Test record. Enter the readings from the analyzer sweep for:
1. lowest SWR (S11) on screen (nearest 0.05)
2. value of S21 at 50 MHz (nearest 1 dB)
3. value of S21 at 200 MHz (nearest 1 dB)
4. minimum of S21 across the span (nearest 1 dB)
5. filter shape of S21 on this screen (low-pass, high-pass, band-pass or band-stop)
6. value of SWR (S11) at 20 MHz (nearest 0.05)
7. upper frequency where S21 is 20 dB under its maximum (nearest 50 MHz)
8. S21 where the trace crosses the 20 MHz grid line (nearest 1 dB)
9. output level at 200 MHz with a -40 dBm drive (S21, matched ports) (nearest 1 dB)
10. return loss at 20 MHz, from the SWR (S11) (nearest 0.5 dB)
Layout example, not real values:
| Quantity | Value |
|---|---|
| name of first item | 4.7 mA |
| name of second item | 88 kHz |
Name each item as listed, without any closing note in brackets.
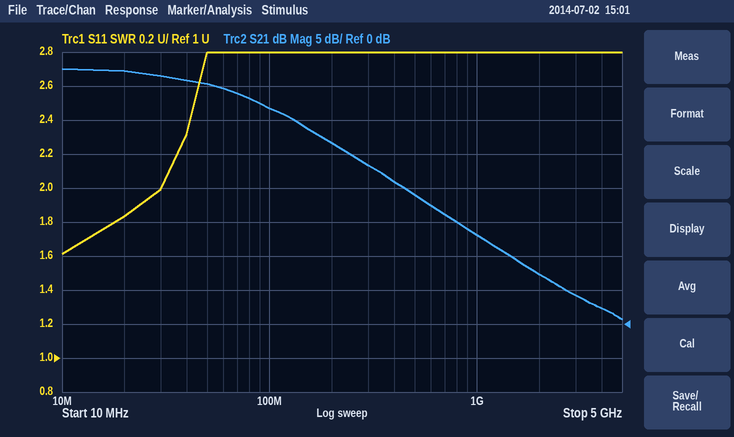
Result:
| Quantity | Value |
|---|---|
| lowest SWR (S11) on screen | 1.60 |
| value of S21 at 50 MHz | 35 dB |
| value of S21 at 200 MHz | 27 dB |
| minimum of S21 across the span | 1 dB |
| filter shape of S21 on this screen | low-pass |
| value of SWR (S11) at 20 MHz | 1.85 |
| upper frequency where S21 is 20 dB under its maximum | 600 MHz |
| S21 where the trace crosses the 20 MHz grid line | 37 dB |
| output level at 200 MHz with a -40 dBm drive (S21, matched ports) | -13 dBm |
| return loss at 20 MHz, from the SWR (S11) | 10.5 dB |
